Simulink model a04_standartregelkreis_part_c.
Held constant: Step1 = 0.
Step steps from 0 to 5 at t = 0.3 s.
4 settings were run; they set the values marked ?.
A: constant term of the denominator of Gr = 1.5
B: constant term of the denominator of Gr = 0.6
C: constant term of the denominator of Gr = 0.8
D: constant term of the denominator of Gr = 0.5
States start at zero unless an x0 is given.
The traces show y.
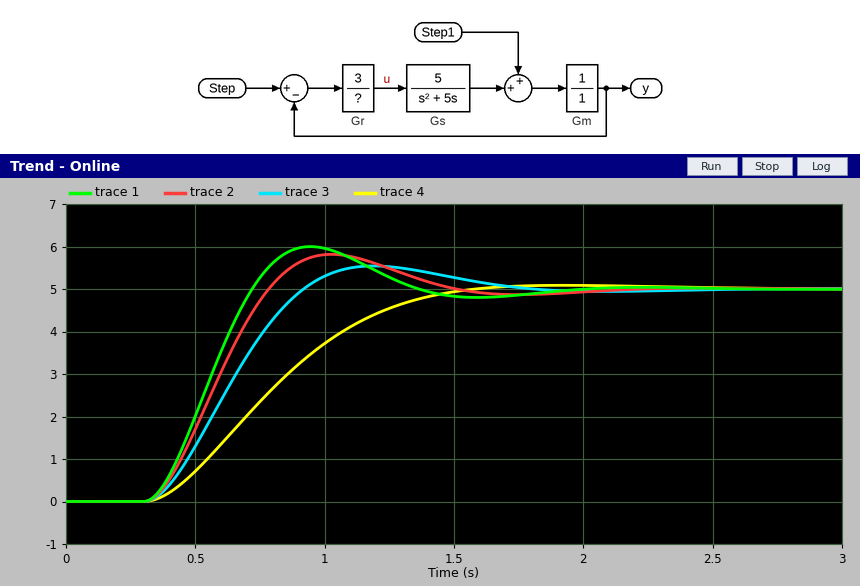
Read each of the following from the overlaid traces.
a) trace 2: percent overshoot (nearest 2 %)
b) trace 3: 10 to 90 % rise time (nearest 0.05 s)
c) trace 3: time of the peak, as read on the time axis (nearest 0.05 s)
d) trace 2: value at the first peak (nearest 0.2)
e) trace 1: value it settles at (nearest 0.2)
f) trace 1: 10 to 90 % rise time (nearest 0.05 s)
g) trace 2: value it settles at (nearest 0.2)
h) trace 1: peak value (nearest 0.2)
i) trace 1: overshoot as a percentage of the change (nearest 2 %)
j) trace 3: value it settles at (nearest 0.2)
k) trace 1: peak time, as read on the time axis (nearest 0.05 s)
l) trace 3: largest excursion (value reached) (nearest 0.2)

16 %
0.40 s
1.20 s
5.8
5.0
0.30 s
5.0
6.0
20 %
5.0
0.95 s
5.6
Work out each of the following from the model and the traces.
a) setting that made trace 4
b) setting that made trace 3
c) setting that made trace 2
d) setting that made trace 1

A
C
B
D
